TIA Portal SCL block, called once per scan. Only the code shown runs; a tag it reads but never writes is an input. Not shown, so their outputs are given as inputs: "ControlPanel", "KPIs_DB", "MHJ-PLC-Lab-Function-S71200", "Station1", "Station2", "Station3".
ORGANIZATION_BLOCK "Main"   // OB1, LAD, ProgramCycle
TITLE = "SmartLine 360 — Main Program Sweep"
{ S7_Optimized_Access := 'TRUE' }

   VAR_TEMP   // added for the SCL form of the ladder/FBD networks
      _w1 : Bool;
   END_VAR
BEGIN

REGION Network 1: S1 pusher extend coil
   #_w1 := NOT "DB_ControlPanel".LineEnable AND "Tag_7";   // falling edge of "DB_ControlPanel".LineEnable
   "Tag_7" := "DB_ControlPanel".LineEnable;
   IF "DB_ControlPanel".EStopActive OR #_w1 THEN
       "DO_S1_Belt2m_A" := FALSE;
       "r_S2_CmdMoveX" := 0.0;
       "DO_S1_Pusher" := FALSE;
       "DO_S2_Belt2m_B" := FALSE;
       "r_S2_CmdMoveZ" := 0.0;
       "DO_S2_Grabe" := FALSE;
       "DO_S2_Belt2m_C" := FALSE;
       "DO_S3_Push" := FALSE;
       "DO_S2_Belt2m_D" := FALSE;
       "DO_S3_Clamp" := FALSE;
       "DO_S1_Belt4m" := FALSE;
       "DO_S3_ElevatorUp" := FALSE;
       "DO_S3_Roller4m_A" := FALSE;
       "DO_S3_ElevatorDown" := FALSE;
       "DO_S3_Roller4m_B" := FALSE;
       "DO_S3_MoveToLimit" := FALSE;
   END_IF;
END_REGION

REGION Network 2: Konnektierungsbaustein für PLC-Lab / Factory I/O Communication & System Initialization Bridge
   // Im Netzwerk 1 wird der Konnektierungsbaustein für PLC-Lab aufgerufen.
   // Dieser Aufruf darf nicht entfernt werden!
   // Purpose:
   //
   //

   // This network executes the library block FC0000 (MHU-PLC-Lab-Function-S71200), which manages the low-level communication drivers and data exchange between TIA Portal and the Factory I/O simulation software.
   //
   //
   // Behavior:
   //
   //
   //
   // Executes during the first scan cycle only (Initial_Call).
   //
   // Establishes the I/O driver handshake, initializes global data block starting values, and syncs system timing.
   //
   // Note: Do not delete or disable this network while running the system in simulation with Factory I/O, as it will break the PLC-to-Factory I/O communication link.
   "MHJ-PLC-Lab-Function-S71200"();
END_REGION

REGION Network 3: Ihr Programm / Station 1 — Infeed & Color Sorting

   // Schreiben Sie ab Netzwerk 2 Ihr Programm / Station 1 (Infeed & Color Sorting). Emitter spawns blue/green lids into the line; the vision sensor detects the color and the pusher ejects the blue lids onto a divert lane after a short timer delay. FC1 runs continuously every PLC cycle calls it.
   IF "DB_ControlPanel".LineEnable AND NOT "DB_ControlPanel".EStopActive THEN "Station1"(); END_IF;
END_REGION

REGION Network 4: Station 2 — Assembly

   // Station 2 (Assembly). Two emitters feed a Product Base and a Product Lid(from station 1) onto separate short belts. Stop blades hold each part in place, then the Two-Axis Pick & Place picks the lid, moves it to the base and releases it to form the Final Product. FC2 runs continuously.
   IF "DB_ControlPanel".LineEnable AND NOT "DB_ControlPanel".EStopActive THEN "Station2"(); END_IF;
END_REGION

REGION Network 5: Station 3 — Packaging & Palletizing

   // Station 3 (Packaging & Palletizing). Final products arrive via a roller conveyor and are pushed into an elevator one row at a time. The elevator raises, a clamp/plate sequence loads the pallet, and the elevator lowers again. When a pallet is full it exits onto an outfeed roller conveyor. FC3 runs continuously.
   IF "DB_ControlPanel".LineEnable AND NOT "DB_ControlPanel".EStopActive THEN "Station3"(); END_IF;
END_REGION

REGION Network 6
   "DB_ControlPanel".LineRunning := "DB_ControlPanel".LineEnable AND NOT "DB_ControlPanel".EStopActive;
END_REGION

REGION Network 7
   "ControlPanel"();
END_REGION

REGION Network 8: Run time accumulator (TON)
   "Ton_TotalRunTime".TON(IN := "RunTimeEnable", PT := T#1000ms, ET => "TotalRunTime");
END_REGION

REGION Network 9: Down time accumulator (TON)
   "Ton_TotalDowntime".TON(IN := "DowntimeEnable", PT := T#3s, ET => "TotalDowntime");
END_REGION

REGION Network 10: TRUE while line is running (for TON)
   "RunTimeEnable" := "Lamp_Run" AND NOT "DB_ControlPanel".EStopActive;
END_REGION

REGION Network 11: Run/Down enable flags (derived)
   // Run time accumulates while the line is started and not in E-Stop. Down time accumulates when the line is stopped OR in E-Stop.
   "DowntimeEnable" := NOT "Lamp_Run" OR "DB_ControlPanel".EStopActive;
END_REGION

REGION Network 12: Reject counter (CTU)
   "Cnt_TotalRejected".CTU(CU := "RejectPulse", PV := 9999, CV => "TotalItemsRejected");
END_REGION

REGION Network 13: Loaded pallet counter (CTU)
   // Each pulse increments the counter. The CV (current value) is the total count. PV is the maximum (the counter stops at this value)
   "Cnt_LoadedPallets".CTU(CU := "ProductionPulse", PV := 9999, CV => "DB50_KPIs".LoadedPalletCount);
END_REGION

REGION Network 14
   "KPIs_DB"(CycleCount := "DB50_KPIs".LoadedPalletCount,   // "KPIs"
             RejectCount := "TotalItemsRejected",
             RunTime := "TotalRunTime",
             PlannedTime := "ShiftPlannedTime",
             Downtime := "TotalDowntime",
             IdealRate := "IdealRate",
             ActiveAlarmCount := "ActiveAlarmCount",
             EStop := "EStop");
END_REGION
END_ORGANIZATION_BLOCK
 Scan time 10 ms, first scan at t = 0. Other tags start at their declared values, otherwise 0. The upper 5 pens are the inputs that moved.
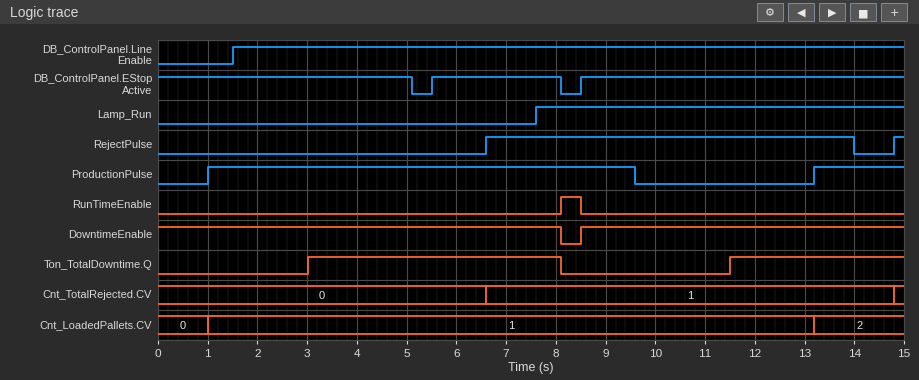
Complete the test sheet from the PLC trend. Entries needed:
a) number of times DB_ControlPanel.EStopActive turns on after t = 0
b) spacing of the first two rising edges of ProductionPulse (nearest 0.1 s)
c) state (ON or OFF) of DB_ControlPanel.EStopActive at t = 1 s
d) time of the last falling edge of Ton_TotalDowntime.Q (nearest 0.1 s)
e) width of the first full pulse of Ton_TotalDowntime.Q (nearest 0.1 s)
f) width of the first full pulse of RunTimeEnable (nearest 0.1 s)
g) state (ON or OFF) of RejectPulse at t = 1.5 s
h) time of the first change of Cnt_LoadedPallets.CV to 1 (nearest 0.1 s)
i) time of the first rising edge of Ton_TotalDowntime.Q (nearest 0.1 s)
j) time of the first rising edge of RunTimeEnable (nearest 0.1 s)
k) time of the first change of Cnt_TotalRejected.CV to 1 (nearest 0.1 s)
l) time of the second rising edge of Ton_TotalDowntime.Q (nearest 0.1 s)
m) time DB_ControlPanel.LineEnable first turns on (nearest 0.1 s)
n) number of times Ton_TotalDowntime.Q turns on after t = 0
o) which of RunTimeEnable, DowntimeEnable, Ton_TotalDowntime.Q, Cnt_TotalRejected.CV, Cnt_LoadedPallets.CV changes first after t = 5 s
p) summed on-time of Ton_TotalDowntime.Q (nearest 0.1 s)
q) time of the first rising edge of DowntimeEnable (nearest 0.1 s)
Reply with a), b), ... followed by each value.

a) 2
b) 12.2 s
c) ON
d) 8.1 s
e) 5.1 s
f) 0.4 s
g) OFF
h) 1.0 s
i) 3.0 s
j) 8.1 s
k) 6.6 s
l) 11.5 s
m) 1.5 s
n) 2
o) Cnt_TotalRejected.CV
p) 8.6 s
q) 8.5 s
